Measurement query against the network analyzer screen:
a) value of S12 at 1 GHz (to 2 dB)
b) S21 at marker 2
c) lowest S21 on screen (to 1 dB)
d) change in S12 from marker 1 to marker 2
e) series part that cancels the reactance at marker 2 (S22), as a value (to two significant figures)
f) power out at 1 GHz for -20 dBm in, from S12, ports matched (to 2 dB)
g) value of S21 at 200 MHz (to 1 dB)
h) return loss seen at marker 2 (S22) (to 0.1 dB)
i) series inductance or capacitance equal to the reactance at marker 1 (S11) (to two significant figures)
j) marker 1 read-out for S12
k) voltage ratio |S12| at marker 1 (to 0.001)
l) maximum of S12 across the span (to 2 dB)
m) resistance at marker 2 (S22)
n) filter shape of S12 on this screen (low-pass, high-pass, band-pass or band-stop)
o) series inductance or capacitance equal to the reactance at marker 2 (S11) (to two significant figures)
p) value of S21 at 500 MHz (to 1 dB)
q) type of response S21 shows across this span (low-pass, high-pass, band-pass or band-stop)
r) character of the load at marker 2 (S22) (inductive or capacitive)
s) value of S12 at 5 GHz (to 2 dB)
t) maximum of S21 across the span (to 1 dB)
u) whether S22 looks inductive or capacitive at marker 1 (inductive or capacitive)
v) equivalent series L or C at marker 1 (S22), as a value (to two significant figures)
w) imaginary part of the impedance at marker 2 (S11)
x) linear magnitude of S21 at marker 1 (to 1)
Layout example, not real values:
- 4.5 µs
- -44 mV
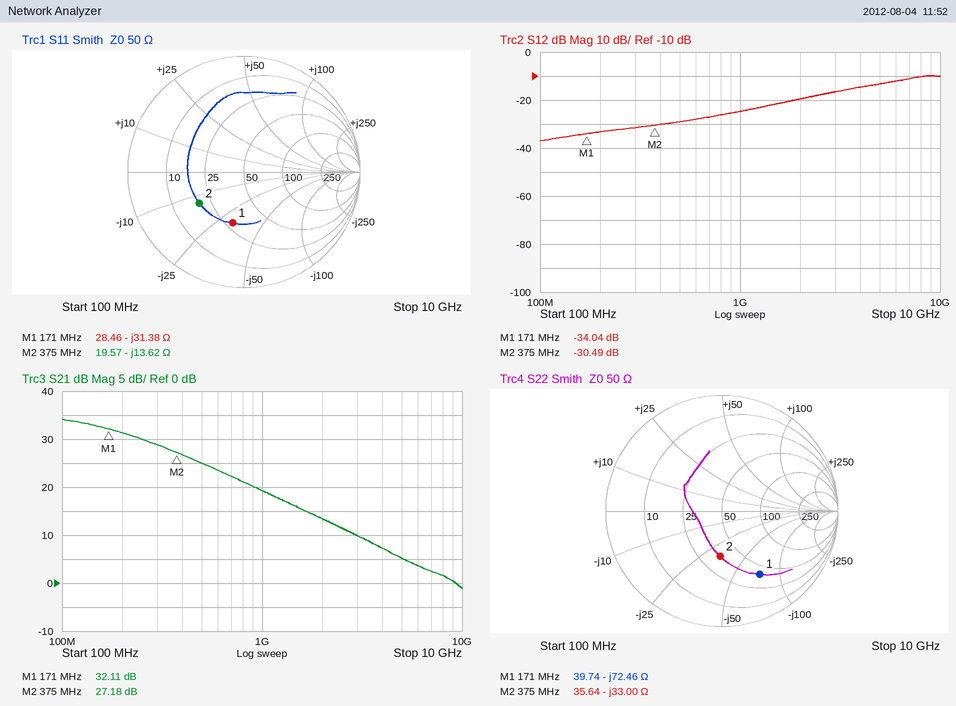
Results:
- -24 dB
- 27.18 dB
- -1 dB
- 3.55 dB
- 14 nH
- -44 dBm
- 31 dB
- 8.1 dB
- 30 pF
- -34.04 dB
- 0.020
- -10 dB
- 35.64 Ω
- high-pass
- 31 pF
- 25 dB
- low-pass
- capacitive
- -14 dB
- 34 dB
- capacitive
- 13 pF
- -13.62 Ω
- 40
